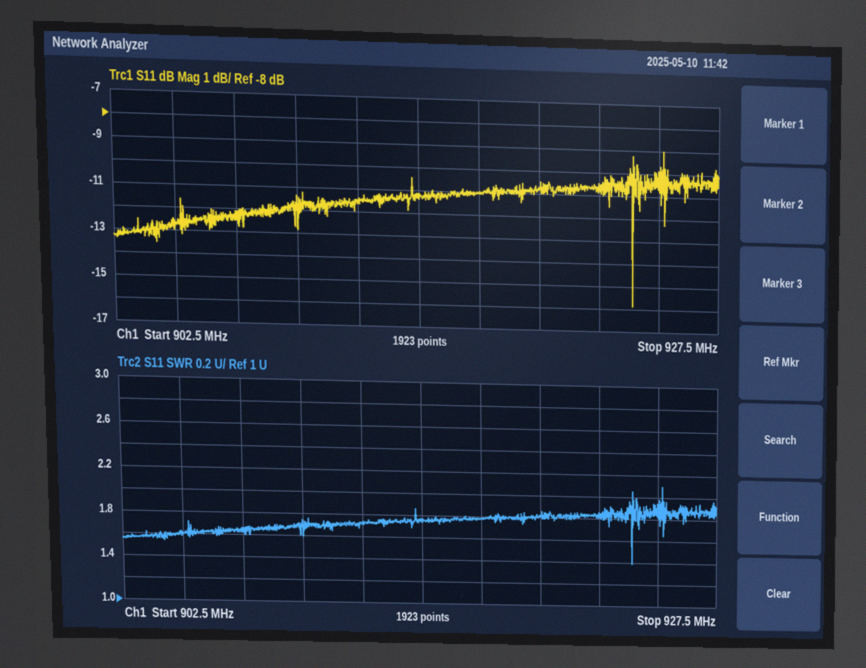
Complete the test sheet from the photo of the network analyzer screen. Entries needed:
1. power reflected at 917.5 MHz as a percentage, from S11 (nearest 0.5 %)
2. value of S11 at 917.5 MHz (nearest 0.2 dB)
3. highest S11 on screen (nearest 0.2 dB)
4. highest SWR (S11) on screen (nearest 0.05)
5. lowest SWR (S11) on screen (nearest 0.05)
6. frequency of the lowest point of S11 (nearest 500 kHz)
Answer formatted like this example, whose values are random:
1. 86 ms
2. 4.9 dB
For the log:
1. 8.0 %
2. -11.0 dB
3. -9.0 dB
4. 2.10
5. 1.40
6. 924.0 MHz
